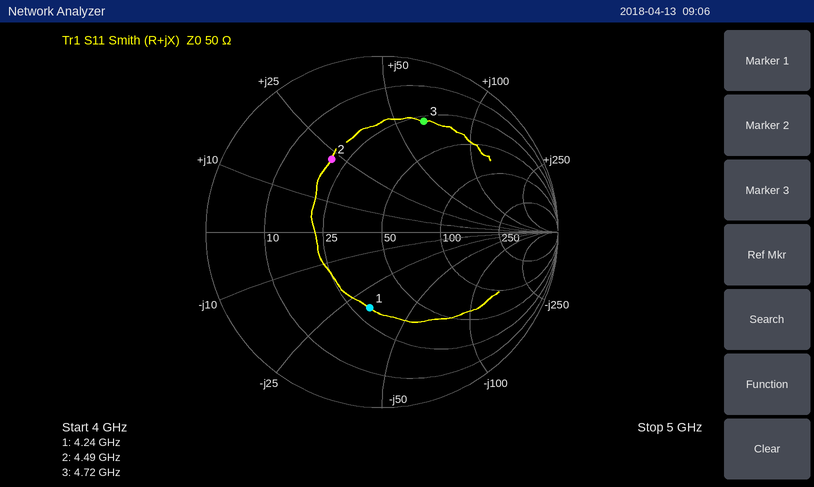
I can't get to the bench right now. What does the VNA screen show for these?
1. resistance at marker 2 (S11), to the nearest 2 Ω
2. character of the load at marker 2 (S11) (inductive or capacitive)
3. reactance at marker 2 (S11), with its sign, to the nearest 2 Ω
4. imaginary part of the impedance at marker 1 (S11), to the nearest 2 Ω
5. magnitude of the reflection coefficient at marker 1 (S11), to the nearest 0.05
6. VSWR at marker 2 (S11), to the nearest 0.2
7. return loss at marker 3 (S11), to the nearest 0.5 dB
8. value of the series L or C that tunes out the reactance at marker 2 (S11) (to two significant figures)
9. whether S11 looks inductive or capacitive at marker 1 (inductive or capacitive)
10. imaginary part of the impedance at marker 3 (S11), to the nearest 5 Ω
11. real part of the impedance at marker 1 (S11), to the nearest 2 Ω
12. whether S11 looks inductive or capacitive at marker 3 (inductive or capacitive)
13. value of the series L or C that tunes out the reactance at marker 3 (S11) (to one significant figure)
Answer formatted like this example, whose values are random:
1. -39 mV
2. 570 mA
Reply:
1. 20 Ω
2. inductive
3. +22 Ω
4. -32 Ω
5. 0.45
6. 3.0
7. 3.5 dB
8. 1.6 pF
9. capacitive
10. +65 Ω
11. 30 Ω
12. inductive
13. 500 fF
